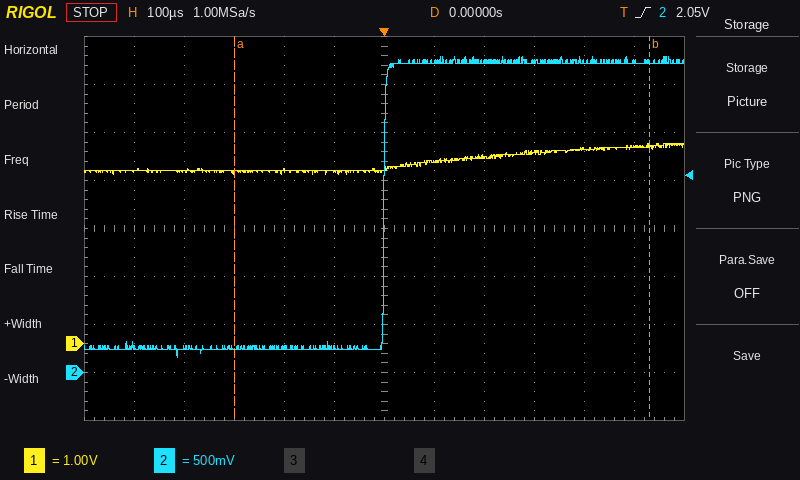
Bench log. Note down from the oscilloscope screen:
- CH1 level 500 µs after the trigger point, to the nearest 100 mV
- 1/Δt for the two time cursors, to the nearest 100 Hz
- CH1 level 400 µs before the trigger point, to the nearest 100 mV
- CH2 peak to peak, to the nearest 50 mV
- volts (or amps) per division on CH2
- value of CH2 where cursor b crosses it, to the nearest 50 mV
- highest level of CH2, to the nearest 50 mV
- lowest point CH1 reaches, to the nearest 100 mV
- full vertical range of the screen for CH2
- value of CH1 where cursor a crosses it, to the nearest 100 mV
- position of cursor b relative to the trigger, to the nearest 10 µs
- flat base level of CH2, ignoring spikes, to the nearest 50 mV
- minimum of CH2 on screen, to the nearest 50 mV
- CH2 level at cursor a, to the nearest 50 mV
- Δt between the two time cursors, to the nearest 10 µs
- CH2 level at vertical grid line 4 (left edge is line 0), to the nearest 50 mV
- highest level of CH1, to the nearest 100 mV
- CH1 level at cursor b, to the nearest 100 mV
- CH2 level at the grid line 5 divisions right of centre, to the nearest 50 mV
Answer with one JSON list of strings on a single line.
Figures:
["4.1 V", "1.2 kHz", "3.6 V", "3.15 V", "500 mV", "3.25 V", "3.30 V", "3.5 V", "4 V", "3.6 V", "+530 µs", "250 mV", "150 mV", "250 mV", "830 µs", "250 mV", "4.2 V", "4.1 V", "3.25 V"]
